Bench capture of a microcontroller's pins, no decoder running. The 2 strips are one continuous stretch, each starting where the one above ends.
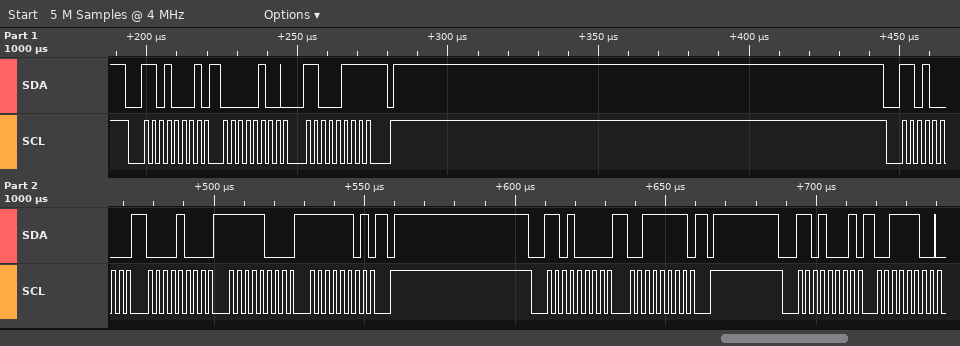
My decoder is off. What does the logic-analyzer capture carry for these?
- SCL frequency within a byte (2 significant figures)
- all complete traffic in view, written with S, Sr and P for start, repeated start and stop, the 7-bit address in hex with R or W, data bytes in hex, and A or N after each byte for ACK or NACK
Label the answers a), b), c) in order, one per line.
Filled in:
a) 400 kHz
b) S 68R A 04 A C7 N P S 68W A 08 A F8 A FD A P S 68W A 3F A P S 68R A 3C A
